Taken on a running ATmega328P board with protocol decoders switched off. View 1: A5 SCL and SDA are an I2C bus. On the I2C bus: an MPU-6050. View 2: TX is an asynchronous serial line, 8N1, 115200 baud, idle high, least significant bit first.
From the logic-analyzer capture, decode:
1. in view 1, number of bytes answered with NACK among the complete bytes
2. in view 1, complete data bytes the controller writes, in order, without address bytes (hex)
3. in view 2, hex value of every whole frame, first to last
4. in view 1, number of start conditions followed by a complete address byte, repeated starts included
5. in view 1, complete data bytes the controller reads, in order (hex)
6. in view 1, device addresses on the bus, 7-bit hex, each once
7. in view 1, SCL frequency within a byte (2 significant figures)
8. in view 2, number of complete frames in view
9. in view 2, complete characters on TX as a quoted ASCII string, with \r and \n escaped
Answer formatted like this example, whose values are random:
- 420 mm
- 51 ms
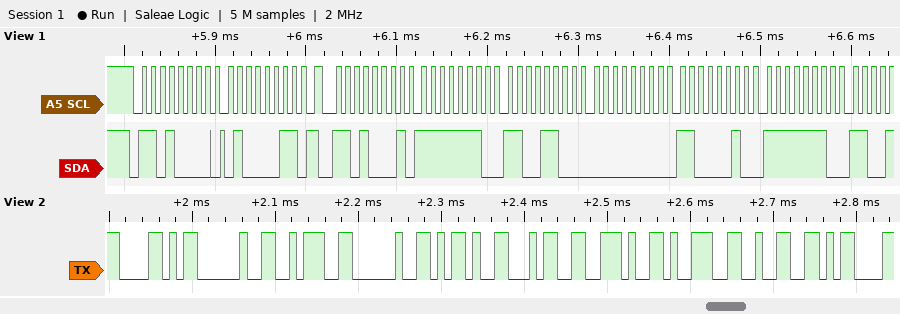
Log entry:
- 0
- 43
- 58 20 3A 20 2D 34 2E 39 32 0D
- 2
- FE CC 00 C2 FE
- 0x68
- 100 kHz
- 10
- "X : -4.92\r"
